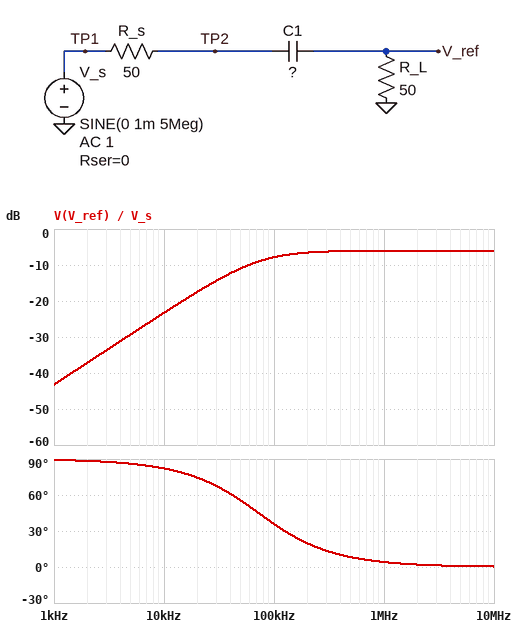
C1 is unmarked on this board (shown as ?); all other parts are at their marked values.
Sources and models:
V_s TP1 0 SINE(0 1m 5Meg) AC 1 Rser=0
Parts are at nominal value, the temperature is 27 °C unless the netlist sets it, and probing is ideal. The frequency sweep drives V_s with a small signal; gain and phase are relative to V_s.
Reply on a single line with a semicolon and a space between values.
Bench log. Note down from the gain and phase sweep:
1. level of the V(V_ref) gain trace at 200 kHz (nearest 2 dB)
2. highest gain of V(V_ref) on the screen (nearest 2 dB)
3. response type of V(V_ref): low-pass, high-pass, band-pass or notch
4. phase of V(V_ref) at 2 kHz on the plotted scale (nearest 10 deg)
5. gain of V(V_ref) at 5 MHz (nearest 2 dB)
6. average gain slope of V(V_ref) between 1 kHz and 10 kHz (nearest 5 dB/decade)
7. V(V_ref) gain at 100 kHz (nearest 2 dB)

-6 dB; -6 dB; high-pass; 90 deg; -6 dB; 20 dB/decade; -8 dB
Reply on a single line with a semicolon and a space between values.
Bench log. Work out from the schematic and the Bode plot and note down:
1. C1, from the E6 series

22 nF
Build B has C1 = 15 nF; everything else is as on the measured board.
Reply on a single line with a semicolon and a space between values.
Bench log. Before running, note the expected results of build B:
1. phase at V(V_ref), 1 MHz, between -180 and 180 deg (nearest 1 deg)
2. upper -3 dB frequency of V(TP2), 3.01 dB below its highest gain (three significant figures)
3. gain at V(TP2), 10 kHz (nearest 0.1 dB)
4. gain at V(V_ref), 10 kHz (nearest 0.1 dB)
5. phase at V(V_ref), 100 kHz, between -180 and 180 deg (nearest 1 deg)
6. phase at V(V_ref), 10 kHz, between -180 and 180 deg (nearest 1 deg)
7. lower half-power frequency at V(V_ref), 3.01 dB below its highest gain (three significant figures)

6 deg; 150 kHz; 0 dB; -26.6 dB; 47 deg; 85 deg; 106 kHz
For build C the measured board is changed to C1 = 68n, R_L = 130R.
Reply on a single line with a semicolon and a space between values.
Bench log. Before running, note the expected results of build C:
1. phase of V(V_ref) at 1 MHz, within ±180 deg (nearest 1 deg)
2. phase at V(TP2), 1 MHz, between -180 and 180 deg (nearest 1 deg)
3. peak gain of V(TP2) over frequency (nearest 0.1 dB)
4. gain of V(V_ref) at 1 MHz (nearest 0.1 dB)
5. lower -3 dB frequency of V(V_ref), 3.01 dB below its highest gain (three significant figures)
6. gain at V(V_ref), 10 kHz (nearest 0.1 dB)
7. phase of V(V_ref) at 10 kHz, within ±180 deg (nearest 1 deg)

1 deg; 0 deg; 0 dB; -2.8 dB; 13.0 kHz; -7.1 dB; 52 deg
